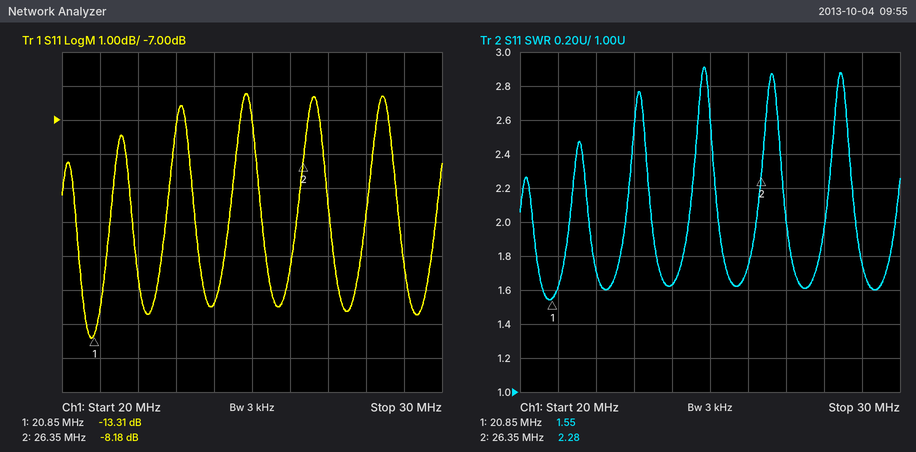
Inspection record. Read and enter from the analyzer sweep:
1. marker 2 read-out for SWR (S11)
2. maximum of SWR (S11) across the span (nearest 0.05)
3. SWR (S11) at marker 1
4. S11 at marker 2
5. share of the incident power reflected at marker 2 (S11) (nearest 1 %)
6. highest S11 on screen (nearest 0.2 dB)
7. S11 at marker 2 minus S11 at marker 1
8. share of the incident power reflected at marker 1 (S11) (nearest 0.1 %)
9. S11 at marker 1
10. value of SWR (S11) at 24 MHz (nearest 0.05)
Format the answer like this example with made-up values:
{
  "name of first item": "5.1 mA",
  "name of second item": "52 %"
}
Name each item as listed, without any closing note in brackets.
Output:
{
  "marker 2 read-out for SWR": "2.28",
  "maximum of SWR (S11) across the span": "2.90",
  "SWR (S11) at marker 1": "1.55",
  "S11 at marker 2": "-8.18 dB",
  "share of the incident power reflected at marker 2 (S11)": "15 %",
  "highest S11 on screen": "-6.2 dB",
  "S11 at marker 2 minus S11 at marker 1": "5.13 dB",
  "share of the incident power reflected at marker 1 (S11)": "4.7 %",
  "S11 at marker 1": "-13.31 dB",
  "value of SWR (S11) at 24 MHz": "1.65"
}
